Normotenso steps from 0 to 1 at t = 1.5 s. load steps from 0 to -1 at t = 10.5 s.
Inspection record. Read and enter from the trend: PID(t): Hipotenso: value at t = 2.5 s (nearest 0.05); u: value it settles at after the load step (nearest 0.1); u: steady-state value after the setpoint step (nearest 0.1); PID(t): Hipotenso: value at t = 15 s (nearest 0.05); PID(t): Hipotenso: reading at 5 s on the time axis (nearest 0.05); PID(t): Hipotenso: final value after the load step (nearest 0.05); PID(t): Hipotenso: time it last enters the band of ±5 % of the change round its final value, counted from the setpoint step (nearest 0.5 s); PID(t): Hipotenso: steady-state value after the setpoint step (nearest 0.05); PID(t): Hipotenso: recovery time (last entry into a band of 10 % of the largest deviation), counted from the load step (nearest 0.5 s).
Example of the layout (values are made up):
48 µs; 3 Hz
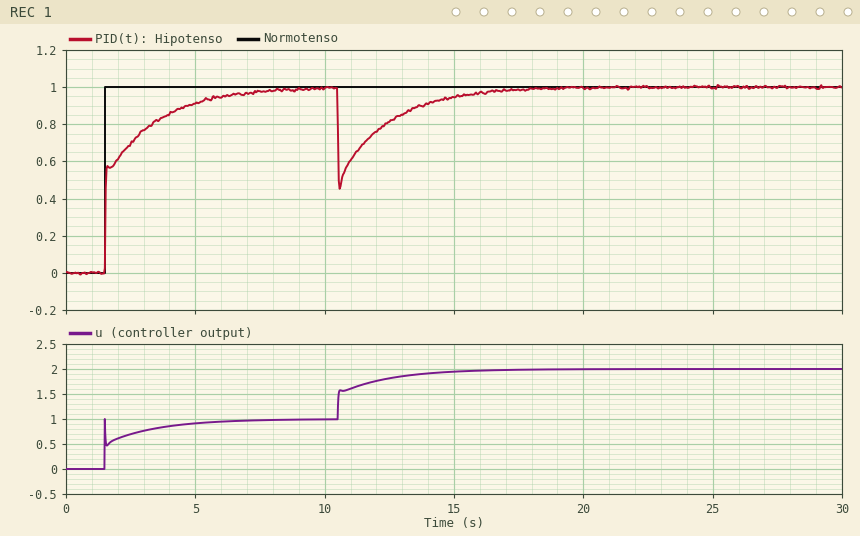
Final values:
0.70; 2.0; 1.0; 0.95; 0.90; 1.00; 4.5 s; 1.00; 4.5 s
